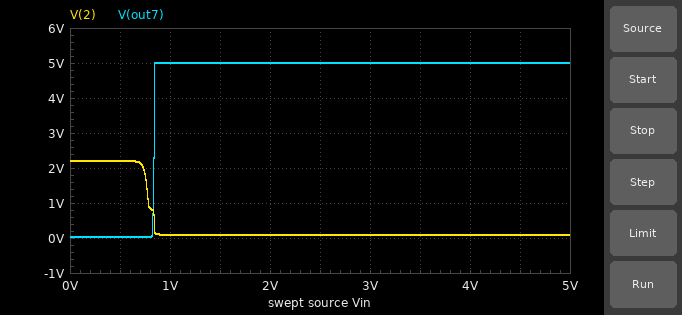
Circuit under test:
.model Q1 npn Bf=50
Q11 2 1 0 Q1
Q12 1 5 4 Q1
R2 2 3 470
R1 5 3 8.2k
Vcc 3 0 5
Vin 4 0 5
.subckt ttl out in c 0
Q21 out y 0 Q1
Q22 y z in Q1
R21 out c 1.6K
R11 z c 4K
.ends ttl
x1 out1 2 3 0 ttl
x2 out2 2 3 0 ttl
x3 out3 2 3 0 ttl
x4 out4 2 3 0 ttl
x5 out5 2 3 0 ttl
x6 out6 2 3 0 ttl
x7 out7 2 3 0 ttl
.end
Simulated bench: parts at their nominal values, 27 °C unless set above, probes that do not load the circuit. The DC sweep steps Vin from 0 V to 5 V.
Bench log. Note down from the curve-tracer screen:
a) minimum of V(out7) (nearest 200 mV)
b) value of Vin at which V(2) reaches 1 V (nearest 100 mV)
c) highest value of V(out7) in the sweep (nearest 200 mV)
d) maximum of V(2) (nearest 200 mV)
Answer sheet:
0 V
800 mV
5.0 V
2.2 V
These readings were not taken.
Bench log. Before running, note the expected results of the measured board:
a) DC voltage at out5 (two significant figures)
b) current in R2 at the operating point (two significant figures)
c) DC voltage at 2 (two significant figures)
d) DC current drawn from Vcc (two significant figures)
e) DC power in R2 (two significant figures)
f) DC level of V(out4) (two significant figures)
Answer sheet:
5.0 V
10 mA
96 mV
18 mA
51 mW
5.0 V
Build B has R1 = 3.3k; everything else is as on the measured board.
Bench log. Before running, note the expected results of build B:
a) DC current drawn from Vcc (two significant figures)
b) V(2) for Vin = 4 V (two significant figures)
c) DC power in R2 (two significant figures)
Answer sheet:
19 mA
66 mV
52 mW
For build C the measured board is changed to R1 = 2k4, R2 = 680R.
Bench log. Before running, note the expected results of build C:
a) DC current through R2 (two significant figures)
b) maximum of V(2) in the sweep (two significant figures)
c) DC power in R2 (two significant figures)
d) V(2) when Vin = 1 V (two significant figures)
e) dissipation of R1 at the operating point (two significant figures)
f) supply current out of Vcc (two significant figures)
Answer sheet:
7.3 mA
960 mV
36 mW
54 mV
4.7 mW
16 mA
